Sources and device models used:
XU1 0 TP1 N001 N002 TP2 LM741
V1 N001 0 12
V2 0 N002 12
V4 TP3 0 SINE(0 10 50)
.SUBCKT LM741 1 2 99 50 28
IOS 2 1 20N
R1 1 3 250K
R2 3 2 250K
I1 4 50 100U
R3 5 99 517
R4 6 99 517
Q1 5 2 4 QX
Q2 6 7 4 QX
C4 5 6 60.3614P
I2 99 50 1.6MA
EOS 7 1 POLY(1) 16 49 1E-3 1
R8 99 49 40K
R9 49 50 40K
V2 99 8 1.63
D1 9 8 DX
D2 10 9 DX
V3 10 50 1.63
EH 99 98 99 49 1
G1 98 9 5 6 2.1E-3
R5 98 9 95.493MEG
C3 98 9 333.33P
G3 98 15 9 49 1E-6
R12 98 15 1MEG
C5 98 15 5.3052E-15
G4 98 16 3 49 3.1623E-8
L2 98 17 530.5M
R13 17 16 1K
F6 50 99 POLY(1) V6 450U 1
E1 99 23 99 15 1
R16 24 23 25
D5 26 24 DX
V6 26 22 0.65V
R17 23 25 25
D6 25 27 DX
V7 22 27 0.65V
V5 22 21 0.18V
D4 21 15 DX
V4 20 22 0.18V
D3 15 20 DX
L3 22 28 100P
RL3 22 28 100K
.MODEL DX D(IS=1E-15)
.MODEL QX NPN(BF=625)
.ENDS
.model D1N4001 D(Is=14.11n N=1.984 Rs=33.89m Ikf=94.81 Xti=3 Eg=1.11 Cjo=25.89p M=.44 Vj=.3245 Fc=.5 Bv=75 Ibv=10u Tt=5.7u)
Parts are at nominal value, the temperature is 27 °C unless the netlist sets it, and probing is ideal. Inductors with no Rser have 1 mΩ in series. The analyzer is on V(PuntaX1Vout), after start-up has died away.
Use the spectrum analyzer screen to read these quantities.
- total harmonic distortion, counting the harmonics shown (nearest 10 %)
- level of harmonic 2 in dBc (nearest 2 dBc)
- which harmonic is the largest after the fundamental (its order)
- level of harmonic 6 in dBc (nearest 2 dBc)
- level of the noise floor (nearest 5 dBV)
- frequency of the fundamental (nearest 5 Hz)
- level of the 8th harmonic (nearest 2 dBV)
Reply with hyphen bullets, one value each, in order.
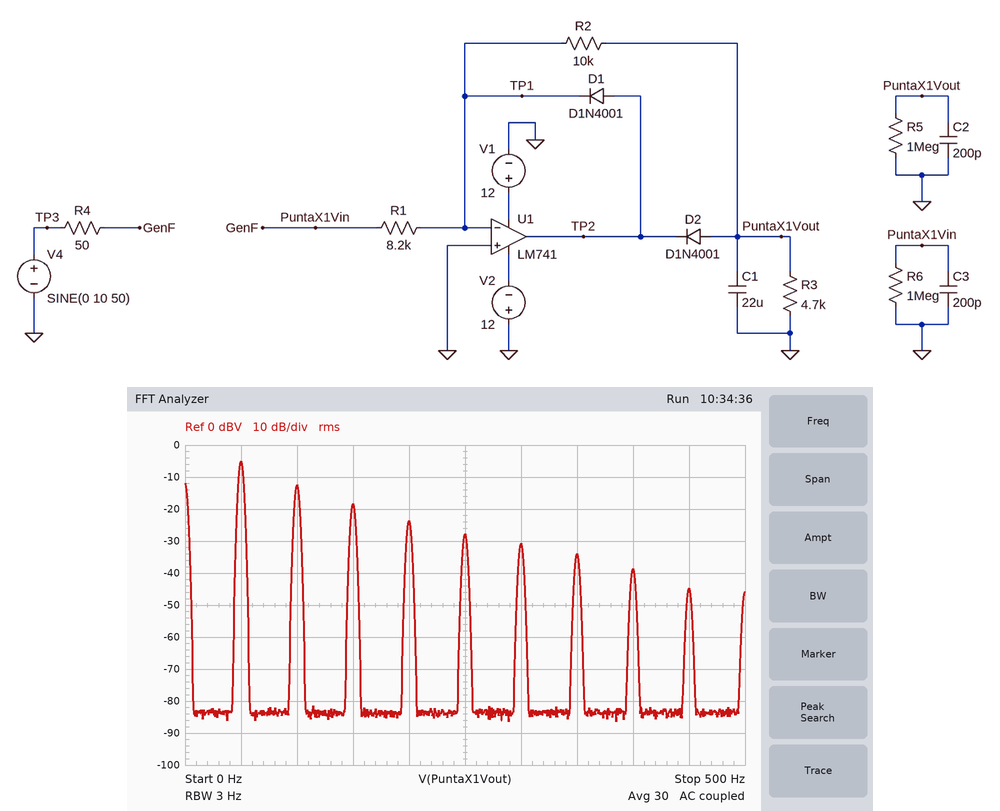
- 50 %
- -8 dBc
- 2
- -26 dBc
- -85 dBV
- 50 Hz
- -38 dBV
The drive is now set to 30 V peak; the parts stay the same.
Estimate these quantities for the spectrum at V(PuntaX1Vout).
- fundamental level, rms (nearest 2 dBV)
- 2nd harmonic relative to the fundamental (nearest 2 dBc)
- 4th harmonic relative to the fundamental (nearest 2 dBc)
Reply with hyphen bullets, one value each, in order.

- -6 dBV
- -10 dBc
- -18 dBc
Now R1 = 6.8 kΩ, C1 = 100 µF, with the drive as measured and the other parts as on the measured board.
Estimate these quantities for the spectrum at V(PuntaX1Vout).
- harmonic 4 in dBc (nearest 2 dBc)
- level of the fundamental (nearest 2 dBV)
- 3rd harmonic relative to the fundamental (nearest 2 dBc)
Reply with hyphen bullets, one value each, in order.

- -26 dBc
- -18 dBV
- -18 dBc
